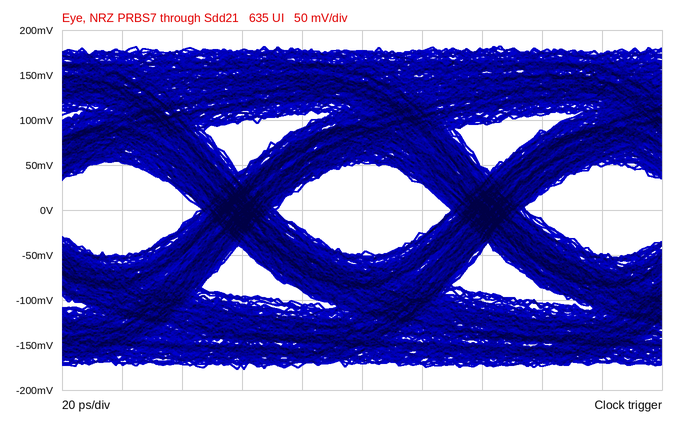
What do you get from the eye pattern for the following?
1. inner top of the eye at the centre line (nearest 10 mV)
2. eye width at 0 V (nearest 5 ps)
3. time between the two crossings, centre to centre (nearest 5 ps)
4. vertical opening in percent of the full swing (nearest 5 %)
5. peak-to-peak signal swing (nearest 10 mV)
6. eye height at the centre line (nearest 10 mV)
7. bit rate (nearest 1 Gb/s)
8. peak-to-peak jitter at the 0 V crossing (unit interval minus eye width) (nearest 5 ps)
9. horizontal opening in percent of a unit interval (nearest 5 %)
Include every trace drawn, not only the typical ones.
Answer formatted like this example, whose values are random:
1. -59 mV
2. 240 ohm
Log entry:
1. 50 mV
2. 60 ps
3. 85 ps
4. 30 %
5. 360 mV
6. 100 mV
7. 12 Gb/s
8. 25 ps
9. 70 %
